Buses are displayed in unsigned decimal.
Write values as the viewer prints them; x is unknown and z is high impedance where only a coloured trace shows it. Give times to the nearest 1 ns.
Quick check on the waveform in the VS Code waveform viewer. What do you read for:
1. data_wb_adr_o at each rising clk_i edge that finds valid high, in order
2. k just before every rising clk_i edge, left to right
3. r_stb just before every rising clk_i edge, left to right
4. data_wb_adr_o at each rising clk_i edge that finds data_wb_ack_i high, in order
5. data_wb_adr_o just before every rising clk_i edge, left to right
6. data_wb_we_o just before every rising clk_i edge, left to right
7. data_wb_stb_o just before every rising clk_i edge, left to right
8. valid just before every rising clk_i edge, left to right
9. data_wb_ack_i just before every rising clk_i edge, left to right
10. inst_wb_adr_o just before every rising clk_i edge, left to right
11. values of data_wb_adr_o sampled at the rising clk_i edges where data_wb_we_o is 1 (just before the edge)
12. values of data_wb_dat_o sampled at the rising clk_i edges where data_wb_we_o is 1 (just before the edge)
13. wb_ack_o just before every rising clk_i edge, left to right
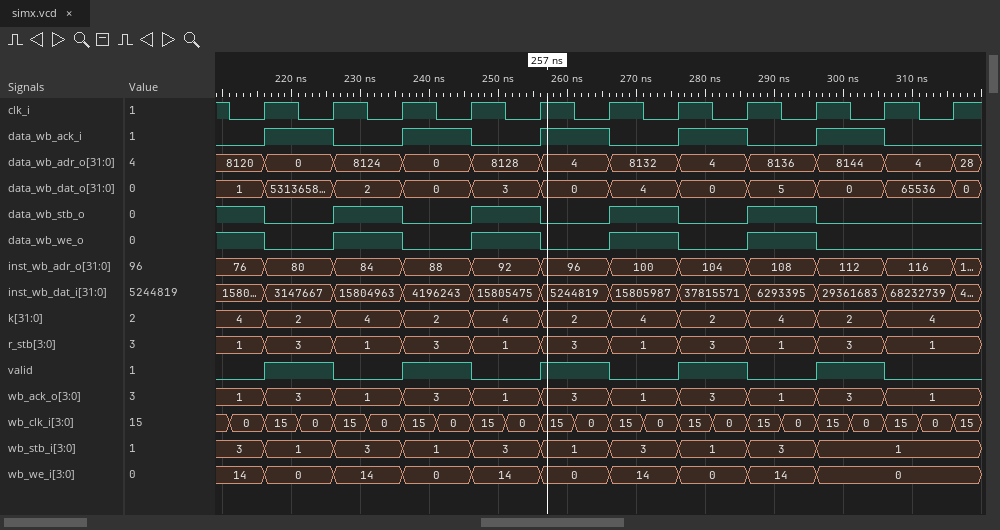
0, 0, 4, 4, 8144
4, 2, 4, 2, 4, 2, 4, 2, 4, 2, 4
1, 3, 1, 3, 1, 3, 1, 3, 1, 3, 1
0, 0, 4, 4, 8144
8120, 0, 8124, 0, 8128, 4, 8132, 4, 8136, 8144, 4
1 0 1 0 1 0 1 0 1 0 0
1 0 1 0 1 0 1 0 1 0 0
0 1 0 1 0 1 0 1 0 1 0
0 1 0 1 0 1 0 1 0 1 0
76, 80, 84, 88, 92, 96, 100, 104, 108, 112, 116
8120, 8124, 8128, 8132, 8136
1, 2, 3, 4, 5
1, 3, 1, 3, 1, 3, 1, 3, 1, 3, 1
